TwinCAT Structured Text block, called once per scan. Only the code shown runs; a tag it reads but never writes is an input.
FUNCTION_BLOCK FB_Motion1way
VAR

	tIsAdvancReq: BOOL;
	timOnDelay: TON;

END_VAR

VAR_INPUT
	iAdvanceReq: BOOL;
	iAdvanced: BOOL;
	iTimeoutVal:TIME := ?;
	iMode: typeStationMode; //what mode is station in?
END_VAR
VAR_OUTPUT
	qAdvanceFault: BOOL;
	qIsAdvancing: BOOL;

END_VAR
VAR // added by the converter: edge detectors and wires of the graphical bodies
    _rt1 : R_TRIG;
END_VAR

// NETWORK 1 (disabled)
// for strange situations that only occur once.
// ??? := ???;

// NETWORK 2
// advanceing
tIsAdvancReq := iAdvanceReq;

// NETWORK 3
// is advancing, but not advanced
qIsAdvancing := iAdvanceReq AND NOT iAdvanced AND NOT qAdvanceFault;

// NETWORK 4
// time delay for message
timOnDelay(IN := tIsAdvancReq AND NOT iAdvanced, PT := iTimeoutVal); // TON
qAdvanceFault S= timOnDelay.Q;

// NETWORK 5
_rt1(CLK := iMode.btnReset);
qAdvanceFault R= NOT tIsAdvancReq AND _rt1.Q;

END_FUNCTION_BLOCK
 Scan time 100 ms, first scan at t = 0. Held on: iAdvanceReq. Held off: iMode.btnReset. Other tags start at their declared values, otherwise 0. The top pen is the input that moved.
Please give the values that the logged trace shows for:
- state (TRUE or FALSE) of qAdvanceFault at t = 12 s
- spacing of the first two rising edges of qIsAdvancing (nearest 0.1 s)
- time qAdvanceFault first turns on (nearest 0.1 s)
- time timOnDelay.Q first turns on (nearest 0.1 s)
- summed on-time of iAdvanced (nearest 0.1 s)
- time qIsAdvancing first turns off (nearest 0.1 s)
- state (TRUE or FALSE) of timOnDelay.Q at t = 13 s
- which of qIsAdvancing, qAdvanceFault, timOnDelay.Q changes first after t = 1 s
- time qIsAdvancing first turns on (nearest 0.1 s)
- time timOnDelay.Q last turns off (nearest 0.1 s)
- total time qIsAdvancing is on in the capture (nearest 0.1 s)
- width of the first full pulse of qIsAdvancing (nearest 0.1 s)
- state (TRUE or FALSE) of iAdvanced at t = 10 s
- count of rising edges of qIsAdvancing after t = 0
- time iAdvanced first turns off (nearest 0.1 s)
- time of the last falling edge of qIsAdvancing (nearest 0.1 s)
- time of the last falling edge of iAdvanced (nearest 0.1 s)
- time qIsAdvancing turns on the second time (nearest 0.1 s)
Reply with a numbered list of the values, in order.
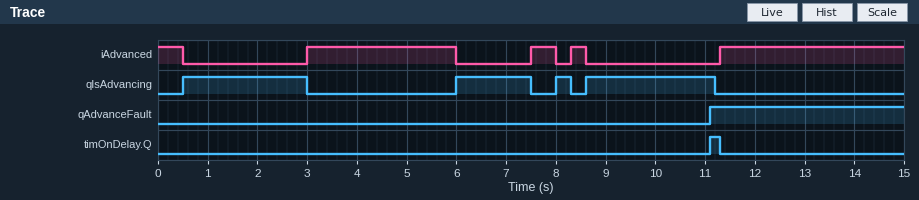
1. TRUE
2. 5.5 s
3. 11.1 s
4. 11.1 s
5. 8.0 s
6. 3.0 s
7. FALSE
8. qIsAdvancing
9. 0.5 s
10. 11.3 s
11. 6.9 s
12. 2.5 s
13. FALSE
14. 4
15. 0.5 s
16. 11.2 s
17. 8.6 s
18. 6.0 s
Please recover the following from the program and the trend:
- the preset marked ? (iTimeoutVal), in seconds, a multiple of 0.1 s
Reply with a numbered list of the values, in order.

1. 2.5 s
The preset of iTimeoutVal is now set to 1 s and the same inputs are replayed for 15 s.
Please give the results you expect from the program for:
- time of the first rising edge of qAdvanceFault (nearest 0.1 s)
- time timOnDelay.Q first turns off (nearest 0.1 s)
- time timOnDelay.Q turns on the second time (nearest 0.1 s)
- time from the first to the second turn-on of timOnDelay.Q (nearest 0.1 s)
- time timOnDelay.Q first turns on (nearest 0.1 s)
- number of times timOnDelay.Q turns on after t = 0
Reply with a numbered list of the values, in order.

1. 1.5 s
2. 3.0 s
3. 7.0 s
4. 5.5 s
5. 1.5 s
6. 3
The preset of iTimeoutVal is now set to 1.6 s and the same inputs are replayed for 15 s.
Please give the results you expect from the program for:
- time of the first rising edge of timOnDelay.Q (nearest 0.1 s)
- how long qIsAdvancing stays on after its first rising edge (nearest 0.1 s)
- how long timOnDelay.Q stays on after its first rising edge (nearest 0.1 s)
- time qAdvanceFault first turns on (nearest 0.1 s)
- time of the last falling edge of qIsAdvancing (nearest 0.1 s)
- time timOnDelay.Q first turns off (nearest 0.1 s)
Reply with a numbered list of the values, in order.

1. 2.1 s
2. 1.7 s
3. 0.9 s
4. 2.1 s
5. 2.2 s
6. 3.0 s
